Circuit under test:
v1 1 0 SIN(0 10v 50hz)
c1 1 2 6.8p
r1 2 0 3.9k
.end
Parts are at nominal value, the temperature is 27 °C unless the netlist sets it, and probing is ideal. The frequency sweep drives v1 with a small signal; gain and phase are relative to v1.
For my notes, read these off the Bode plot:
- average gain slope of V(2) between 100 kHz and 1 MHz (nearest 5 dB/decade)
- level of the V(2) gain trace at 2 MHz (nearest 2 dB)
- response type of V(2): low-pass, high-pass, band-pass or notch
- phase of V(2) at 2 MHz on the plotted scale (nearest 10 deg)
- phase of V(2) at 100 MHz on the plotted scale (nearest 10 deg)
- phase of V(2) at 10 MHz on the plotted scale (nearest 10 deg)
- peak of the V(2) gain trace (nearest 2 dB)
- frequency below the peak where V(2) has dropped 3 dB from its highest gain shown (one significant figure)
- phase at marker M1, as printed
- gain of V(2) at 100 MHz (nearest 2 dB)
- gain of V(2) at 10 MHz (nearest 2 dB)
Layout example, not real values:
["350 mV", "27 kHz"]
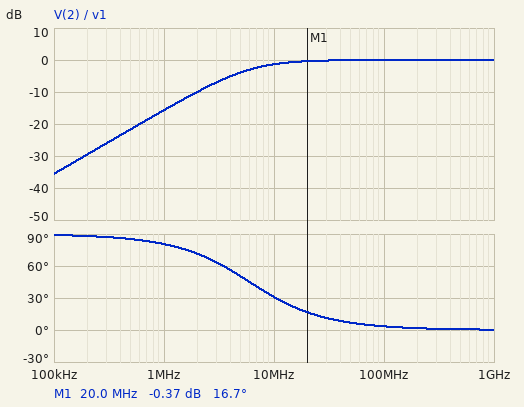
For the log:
["20 dB/decade", "-10 dB", "high-pass", "70 deg", "0 deg", "30 deg", "0 dB", "6 MHz", "16.7 deg", "0 dB", "-2 dB"]
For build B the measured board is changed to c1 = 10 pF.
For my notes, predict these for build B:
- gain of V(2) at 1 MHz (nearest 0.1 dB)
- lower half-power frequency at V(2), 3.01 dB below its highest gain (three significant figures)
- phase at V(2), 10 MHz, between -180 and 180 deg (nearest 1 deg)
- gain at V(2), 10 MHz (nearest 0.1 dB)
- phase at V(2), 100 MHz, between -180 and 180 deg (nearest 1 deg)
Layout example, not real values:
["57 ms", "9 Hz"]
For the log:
["-12.5 dB", "4.08 MHz", "22 deg", "-0.7 dB", "2 deg"]
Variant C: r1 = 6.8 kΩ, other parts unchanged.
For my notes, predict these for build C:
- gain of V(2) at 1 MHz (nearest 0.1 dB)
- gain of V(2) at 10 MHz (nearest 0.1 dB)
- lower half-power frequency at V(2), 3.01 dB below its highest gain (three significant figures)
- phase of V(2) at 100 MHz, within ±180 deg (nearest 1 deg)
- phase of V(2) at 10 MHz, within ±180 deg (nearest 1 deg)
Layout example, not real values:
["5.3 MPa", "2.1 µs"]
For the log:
["-11.1 dB", "-0.5 dB", "3.44 MHz", "2 deg", "19 deg"]
